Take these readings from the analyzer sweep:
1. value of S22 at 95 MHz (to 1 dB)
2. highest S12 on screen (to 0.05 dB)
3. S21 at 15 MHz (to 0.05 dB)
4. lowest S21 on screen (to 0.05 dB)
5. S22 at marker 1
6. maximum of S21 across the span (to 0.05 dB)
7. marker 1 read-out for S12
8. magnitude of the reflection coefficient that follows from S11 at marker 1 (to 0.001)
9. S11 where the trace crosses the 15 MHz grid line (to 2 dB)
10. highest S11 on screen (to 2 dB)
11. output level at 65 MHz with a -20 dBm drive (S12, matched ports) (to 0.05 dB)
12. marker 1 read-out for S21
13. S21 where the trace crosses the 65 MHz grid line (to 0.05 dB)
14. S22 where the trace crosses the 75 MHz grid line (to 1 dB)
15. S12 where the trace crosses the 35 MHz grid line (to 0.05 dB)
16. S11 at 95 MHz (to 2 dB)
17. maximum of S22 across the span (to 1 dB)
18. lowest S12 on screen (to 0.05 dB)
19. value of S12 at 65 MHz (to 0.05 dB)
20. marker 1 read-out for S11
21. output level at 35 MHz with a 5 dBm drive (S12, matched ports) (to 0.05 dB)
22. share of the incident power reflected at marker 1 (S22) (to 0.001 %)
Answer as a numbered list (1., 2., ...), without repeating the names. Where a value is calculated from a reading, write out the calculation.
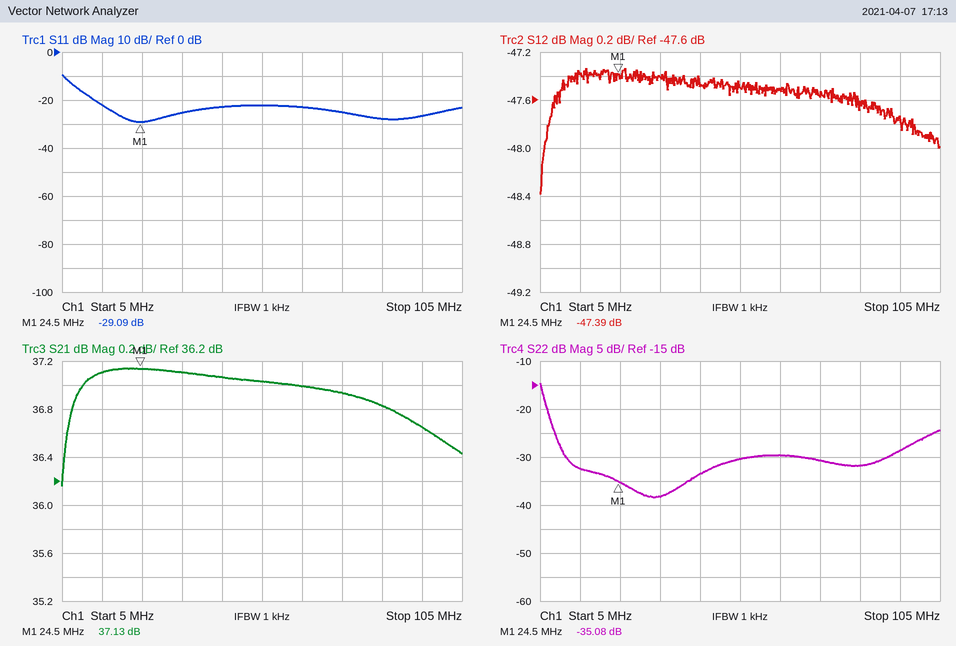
1. -29 dB
2. -47.35 dB
3. 37.10 dB
4. 36.15 dB
5. -35.08 dB
6. 37.15 dB
7. -47.39 dB
8. 10^(-29.09/20) ≈ 0.035
9. -22 dB
10. -10 dB
11. -20 dBm + (-47.50 dB) = -67.50 dBm
12. 37.13 dB
13. 37.00 dB
14. -31 dB
15. -47.40 dB
16. -26 dB
17. -15 dB
18. -48.40 dB
19. -47.50 dB
20. -29.09 dB
21. 5 dBm + (-47.40 dB) = -42.40 dBm
22. 10^(-35.08/10) ≈ 0.031 %
